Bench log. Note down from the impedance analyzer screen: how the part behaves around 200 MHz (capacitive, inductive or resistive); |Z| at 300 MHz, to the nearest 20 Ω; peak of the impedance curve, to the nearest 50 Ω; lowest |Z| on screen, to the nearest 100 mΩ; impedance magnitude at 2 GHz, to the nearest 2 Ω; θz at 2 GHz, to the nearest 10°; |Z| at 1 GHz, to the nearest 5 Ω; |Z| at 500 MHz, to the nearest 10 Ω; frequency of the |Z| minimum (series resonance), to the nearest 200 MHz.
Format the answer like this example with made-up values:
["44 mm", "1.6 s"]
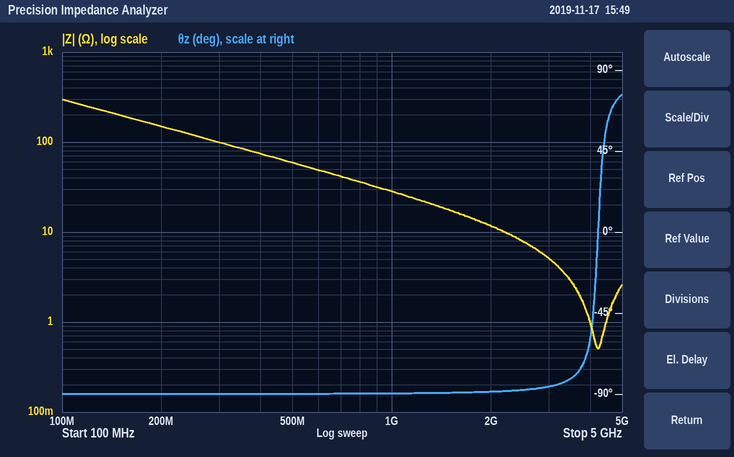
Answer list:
["capacitive", "100 Ω", "300 Ω", "500 mΩ", "12 Ω", "-90°", "30 Ω", "60 Ω", "4.2 GHz"]
